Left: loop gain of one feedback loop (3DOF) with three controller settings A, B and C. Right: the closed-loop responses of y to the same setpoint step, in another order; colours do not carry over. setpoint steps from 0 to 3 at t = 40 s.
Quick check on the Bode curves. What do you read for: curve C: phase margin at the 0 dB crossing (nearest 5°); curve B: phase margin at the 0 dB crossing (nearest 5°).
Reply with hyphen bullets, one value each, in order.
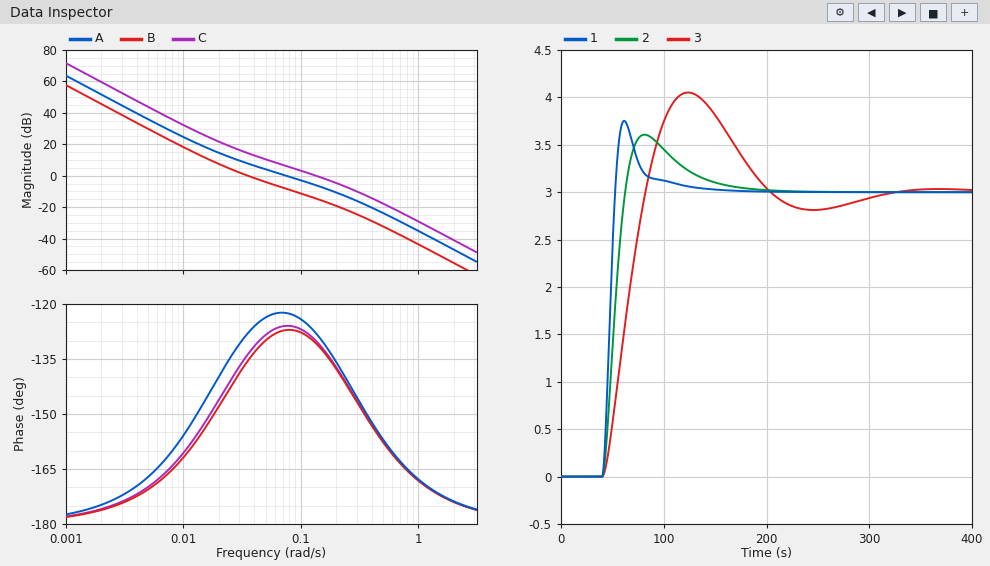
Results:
- 50°
- 45°
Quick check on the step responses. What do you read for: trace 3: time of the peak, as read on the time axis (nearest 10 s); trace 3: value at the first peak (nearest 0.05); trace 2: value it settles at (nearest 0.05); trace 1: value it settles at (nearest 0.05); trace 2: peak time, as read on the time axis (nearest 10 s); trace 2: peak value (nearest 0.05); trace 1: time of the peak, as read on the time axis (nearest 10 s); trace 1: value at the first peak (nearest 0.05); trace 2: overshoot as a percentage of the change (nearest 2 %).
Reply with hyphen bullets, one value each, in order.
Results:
- 120 s
- 4.05
- 3.00
- 3.00
- 80 s
- 3.60
- 60 s
- 3.75
- 20 %
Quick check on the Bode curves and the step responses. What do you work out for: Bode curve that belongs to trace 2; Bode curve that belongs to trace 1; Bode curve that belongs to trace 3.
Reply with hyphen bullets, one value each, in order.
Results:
- A
- C
- B
